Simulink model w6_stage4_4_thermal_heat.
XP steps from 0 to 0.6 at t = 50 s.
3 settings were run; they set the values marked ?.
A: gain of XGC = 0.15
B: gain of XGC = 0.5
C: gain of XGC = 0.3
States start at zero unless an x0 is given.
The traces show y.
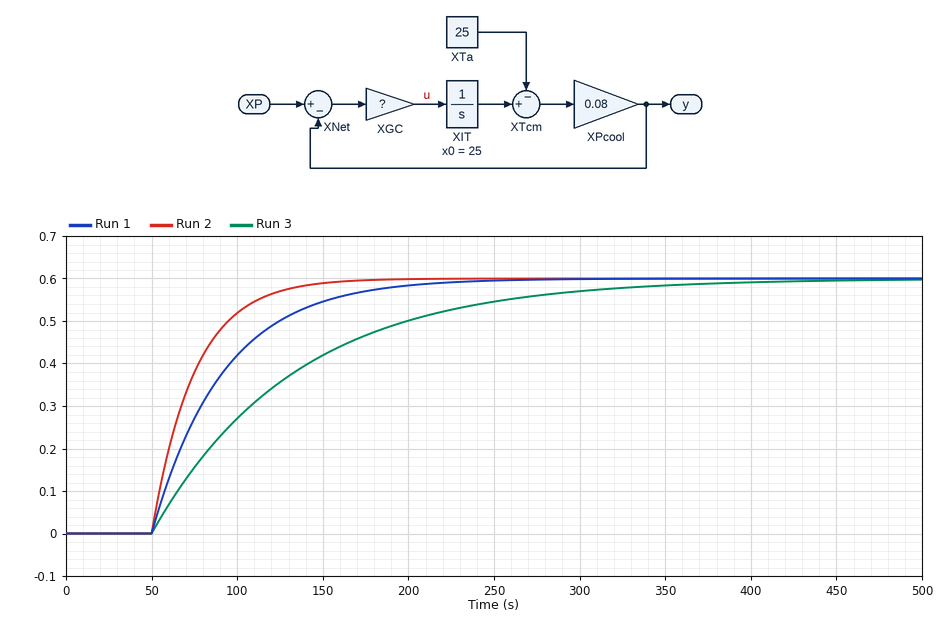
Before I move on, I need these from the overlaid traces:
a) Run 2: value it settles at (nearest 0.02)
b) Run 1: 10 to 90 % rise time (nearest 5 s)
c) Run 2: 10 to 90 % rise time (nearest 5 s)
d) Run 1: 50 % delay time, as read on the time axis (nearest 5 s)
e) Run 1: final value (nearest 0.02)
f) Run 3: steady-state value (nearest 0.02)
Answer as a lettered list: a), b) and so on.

a) 0.60
b) 90 s
c) 55 s
d) 80 s
e) 0.60
f) 0.60
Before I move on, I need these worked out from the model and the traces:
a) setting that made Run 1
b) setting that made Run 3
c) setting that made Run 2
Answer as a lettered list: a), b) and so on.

a) C
b) A
c) B
